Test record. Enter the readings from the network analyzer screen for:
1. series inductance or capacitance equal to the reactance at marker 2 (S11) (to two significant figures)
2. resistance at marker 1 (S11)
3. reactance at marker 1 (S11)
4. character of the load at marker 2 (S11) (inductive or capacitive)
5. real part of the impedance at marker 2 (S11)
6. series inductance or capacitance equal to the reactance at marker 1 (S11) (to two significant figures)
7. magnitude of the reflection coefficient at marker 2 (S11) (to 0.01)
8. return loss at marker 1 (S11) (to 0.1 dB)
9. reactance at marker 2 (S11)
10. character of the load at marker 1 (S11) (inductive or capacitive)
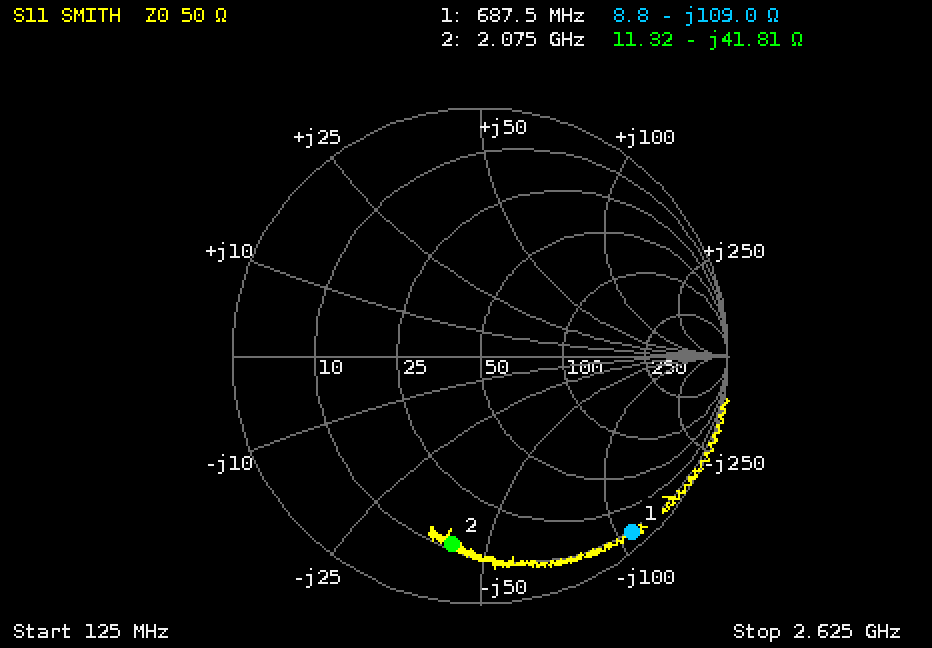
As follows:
1.8 pF
8.8 Ω
-109.0 Ω
capacitive
11.32 Ω
2.1 pF
0.77
0.5 dB
-41.81 Ω
capacitive
